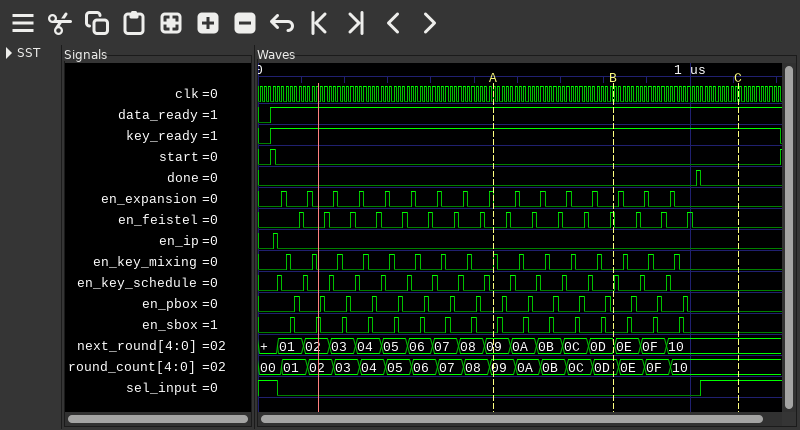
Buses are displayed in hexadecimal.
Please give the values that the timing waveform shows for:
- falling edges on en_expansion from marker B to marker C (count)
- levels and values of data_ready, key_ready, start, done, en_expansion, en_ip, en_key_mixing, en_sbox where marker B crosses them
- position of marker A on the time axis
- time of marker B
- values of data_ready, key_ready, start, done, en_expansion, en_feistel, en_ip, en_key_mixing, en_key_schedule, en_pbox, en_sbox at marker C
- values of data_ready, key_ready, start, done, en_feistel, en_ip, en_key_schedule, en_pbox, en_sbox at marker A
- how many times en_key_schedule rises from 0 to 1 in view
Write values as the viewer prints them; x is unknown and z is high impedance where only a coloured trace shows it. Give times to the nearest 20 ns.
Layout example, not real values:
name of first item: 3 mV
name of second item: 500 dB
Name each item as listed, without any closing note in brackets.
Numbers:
falling edges on en_expansion from marker B to marker C: 3
levels and values of data_ready, key_ready, start, done, en_expansion, en_ip, en_key_mixing, en_sbox where marker B crosses them: data_ready=1, key_ready=1, start=0, done=0, en_expansion=0, en_ip=0, en_key_mixing=0, en_sbox=0
position of marker A on the time axis: 540 ns
time of marker B: 820 ns
values of data_ready, key_ready, start, done, en_expansion, en_feistel, en_ip, en_key_mixing, en_key_schedule, en_pbox, en_sbox at marker C: data_ready=1, key_ready=1, start=0, done=0, en_expansion=0, en_feistel=0, en_ip=0, en_key_mixing=0, en_key_schedule=0, en_pbox=0, en_sbox=0
values of data_ready, key_ready, start, done, en_feistel, en_ip, en_key_schedule, en_pbox, en_sbox at marker A: data_ready=1, key_ready=1, start=0, done=0, en_feistel=0, en_ip=0, en_key_schedule=0, en_pbox=0, en_sbox=0
how many times en_key_schedule rises from 0 to 1 in view: 16
